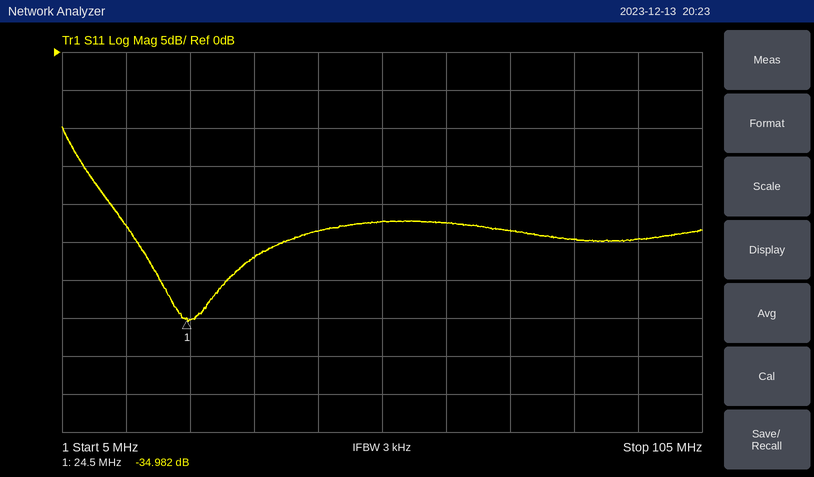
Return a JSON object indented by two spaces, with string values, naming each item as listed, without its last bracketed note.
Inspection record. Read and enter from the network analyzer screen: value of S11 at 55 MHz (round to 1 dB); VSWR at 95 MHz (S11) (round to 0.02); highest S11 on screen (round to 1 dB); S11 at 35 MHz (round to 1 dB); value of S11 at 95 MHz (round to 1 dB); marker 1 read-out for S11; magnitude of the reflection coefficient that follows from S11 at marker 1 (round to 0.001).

{
  "value of S11 at 55 MHz": "-22 dB",
  "VSWR at 95 MHz (S11)": "1.12",
  "highest S11 on screen": "-10 dB",
  "S11 at 35 MHz": "-27 dB",
  "value of S11 at 95 MHz": "-25 dB",
  "marker 1 read-out for S11": "-34.982 dB",
  "magnitude of the reflection coefficient that follows from S11 at marker 1": "0.018"
}
